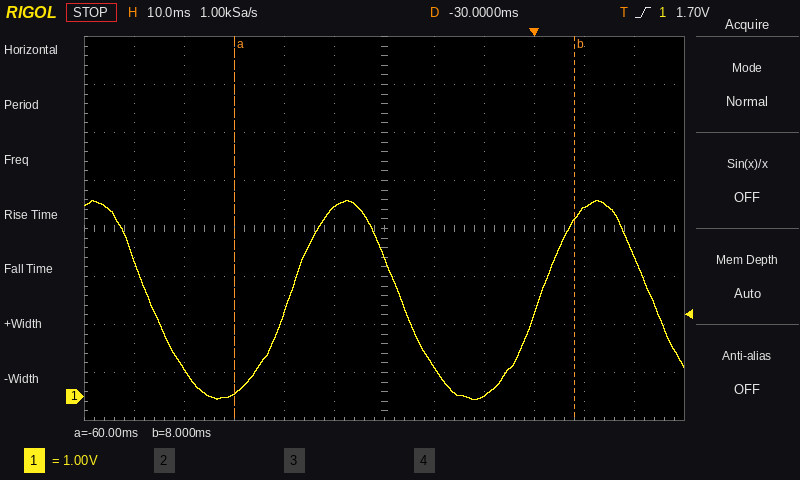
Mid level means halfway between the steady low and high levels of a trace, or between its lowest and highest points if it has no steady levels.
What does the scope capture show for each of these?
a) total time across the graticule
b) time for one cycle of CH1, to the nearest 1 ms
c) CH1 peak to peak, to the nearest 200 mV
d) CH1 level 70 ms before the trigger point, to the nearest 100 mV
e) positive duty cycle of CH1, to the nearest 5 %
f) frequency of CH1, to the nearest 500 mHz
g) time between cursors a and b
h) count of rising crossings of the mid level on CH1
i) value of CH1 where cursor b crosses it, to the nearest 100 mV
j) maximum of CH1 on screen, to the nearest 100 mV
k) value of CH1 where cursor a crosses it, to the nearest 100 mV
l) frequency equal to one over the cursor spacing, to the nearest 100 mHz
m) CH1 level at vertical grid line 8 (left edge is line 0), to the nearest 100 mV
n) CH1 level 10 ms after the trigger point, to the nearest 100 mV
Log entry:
120 ms
50 ms
4.2 V
600 mV
45 %
20.0 Hz
68 ms
2
3.7 V
4.1 V
100 mV
14.7 Hz
0.0 V
3.9 V
